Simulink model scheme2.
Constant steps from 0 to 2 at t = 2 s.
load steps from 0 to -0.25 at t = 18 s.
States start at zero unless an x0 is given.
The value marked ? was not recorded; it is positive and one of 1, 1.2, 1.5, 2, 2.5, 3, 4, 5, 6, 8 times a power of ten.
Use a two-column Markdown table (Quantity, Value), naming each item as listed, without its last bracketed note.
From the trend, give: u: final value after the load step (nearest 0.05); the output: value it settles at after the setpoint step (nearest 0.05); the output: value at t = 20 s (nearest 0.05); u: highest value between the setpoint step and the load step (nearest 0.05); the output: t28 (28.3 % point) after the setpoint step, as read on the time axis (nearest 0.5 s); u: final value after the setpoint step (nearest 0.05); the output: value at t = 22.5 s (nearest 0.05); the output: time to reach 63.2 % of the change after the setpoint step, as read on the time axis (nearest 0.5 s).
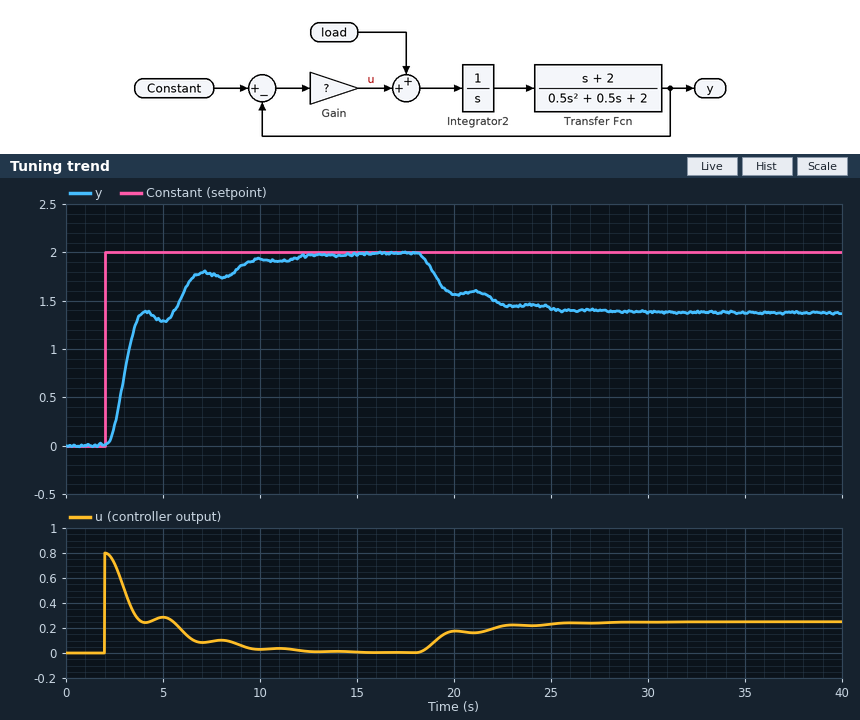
| Quantity | Value |
|---|---|
| u: final value after the load step | 0.25 |
| the output: value it settles at after the setpoint step | 2.00 |
| the output: value at t = 20 s | 1.55 |
| u: highest value between the setpoint step and the load step | 0.80 |
| the output: t28 (28.3 % point) after the setpoint step, as read on the time axis | 3.0 s |
| u: final value after the setpoint step | 0.00 |
| the output: value at t = 22.5 s | 1.45 |
| the output: time to reach 63.2 % of the change after the setpoint step, as read on the time axis | 3.5 s |
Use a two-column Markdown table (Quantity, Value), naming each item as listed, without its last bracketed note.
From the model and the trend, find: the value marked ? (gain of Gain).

| Quantity | Value |
|---|---|
| the value marked ? | 0.4 |
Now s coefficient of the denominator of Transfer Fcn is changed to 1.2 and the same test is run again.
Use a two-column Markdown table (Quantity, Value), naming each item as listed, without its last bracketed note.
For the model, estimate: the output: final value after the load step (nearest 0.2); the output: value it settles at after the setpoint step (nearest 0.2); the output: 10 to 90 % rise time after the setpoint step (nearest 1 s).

| Quantity | Value |
|---|---|
| the output: final value after the load step | 1.4 |
| the output: value it settles at after the setpoint step | 2.0 |
| the output: 10 to 90 % rise time after the setpoint step | 5 s |
